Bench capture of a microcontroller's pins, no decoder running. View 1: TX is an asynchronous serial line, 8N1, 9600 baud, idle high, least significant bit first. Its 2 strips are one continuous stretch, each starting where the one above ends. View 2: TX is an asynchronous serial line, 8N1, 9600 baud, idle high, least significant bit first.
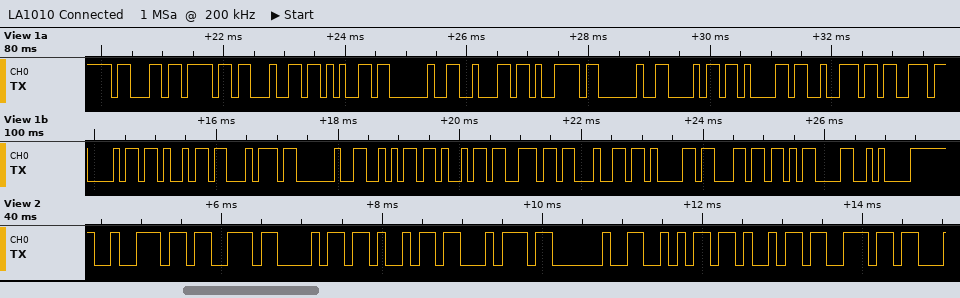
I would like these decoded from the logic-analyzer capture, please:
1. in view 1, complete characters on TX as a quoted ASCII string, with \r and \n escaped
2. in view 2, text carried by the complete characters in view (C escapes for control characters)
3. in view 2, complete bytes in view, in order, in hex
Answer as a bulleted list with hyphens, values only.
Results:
- "code by harshit jindal\r\n"
- "rshit jin"
- 0x72 0x73 0x68 0x69 0x74 0x20 0x6A 0x69 0x6E
